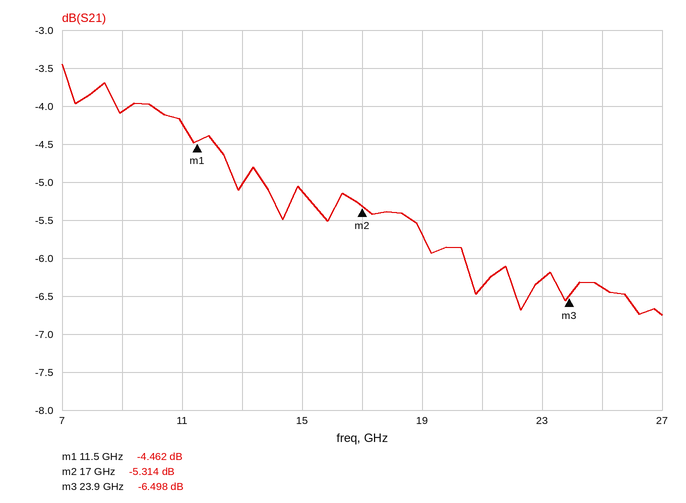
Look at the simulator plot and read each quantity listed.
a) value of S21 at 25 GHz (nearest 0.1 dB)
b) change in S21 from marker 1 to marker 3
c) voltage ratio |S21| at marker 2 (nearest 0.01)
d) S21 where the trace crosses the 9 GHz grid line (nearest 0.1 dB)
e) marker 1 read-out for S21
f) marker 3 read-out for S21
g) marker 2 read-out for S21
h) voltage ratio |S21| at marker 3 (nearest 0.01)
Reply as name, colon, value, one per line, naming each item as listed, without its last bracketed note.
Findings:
value of S21 at 25 GHz: -6.4 dB
change in S21 from marker 1 to marker 3: -2.036 dB
voltage ratio |S21| at marker 2: 0.54
S21 where the trace crosses the 9 GHz grid line: -4.1 dB
marker 1 read-out for S21: -4.462 dB
marker 3 read-out for S21: -6.498 dB
marker 2 read-out for S21: -5.314 dB
voltage ratio |S21| at marker 3: 0.47
